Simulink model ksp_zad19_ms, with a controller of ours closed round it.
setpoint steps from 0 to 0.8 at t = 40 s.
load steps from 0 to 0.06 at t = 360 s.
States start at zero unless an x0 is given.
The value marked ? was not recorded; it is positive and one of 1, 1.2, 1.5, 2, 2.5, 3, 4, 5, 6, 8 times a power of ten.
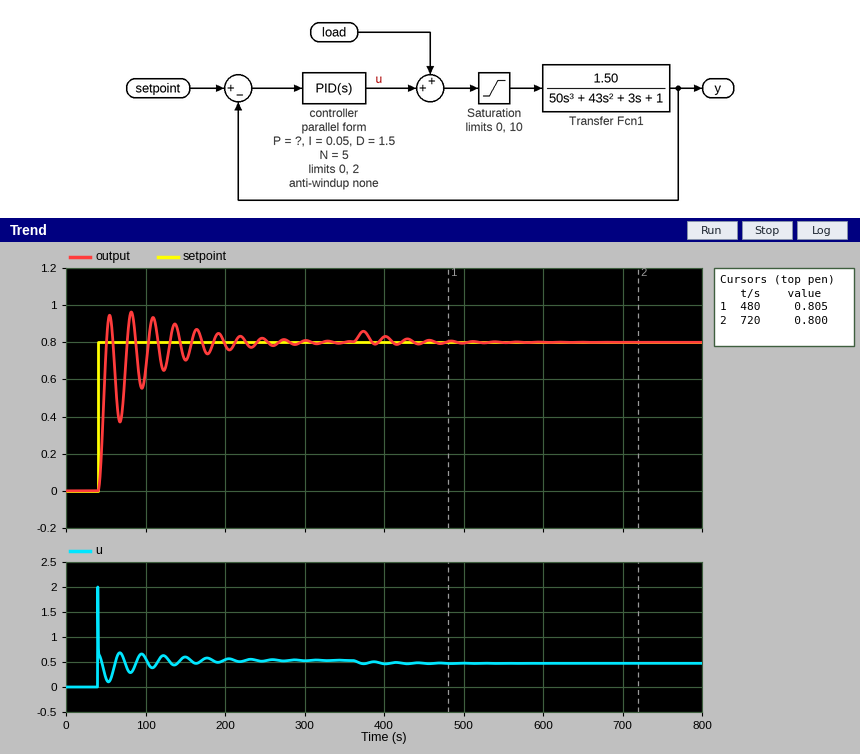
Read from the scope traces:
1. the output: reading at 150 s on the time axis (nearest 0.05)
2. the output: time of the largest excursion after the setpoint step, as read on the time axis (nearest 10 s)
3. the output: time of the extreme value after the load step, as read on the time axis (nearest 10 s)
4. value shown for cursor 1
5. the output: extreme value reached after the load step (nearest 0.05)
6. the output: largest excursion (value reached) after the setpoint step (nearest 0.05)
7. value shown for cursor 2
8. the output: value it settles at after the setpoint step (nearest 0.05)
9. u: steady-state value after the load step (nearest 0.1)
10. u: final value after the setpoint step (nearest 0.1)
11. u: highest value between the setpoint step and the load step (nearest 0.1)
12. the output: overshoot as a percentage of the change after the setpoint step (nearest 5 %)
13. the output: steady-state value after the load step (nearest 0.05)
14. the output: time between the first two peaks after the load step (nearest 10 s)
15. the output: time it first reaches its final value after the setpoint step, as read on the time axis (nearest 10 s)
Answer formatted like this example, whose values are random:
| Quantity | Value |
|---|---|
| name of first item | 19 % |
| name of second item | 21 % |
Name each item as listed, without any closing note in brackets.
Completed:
| Quantity | Value |
|---|---|
| the output: reading at 150 s on the time axis | 0.70 |
| the output: time of the largest excursion after the setpoint step, as read on the time axis | 80 s |
| the output: time of the extreme value after the load step, as read on the time axis | 370 s |
| value shown for cursor 1 | 0.805 |
| the output: extreme value reached after the load step | 0.85 |
| the output: largest excursion (value reached) after the setpoint step | 0.95 |
| value shown for cursor 2 | 0.800 |
| the output: value it settles at after the setpoint step | 0.80 |
| u: steady-state value after the load step | 0.5 |
| u: final value after the setpoint step | 0.5 |
| u: highest value between the setpoint step and the load step | 2.0 |
| the output: overshoot as a percentage of the change after the setpoint step | 20 % |
| the output: steady-state value after the load step | 0.80 |
| the output: time between the first two peaks after the load step | 30 s |
| the output: time it first reaches its final value after the setpoint step, as read on the time axis | 50 s |
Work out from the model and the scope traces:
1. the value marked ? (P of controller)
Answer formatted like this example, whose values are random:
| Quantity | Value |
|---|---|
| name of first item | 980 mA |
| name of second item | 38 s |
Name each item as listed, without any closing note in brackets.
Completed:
| Quantity | Value |
|---|---|
| the value marked ? | 0.8 |
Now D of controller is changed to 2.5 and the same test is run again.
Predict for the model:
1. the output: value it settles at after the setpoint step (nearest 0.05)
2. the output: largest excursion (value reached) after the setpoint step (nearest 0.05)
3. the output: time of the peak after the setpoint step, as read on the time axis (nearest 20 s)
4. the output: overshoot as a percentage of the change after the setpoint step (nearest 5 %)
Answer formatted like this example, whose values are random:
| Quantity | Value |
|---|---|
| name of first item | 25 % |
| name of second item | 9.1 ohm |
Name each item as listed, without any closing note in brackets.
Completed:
| Quantity | Value |
|---|---|
| the output: value it settles at after the setpoint step | 0.80 |
| the output: largest excursion (value reached) after the setpoint step | 0.85 |
| the output: time of the peak after the setpoint step, as read on the time axis | 60 s |
| the output: overshoot as a percentage of the change after the setpoint step | 10 % |
